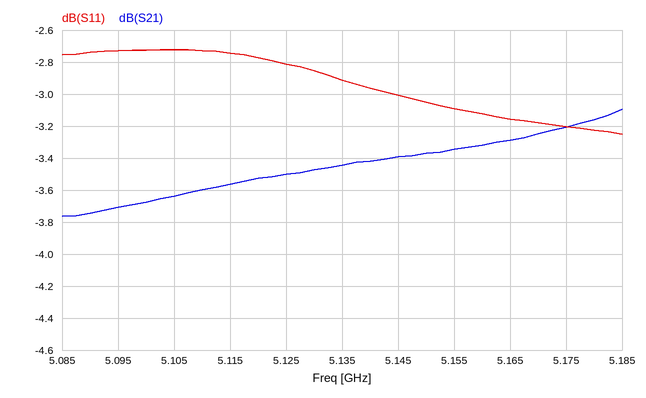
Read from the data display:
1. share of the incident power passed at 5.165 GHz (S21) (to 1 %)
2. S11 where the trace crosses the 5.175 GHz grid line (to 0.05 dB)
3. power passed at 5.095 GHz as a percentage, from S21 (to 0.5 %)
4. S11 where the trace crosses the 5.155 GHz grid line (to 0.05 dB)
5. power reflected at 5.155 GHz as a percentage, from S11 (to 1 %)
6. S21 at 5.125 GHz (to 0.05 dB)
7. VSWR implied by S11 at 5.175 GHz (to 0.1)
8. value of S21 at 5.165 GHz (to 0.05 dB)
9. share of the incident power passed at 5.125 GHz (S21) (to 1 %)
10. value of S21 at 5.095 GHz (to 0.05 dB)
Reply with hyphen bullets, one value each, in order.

- 47 %
- -3.20 dB
- 42.5 %
- -3.10 dB
- 49 %
- -3.50 dB
- 5.5
- -3.30 dB
- 45 %
- -3.70 dB
